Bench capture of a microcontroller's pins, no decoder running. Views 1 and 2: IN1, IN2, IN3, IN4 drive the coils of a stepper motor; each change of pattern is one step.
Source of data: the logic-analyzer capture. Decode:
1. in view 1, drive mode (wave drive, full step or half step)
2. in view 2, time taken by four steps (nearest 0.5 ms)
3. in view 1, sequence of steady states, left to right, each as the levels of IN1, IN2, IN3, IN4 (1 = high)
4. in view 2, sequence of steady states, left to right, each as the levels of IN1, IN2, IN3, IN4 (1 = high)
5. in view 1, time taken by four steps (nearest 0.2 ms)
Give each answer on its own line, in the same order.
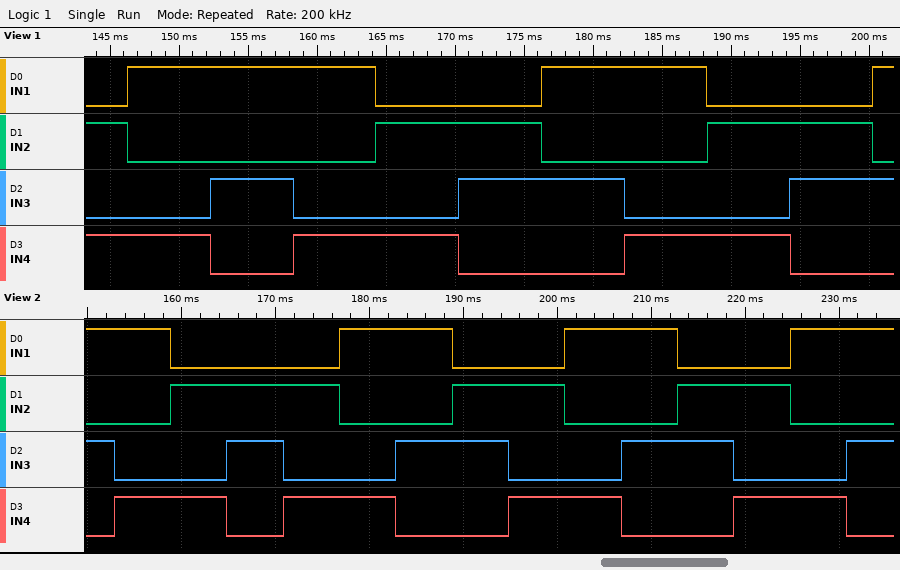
full step
24.0 ms
0101 1001 1010 1001 0101 0110 1010 1001 0101 0110 1010
1010 1001 0101 0110 0101 1001 1010 0110 0101 1001 1010 0110 0101 1001 1010
24.0 ms
